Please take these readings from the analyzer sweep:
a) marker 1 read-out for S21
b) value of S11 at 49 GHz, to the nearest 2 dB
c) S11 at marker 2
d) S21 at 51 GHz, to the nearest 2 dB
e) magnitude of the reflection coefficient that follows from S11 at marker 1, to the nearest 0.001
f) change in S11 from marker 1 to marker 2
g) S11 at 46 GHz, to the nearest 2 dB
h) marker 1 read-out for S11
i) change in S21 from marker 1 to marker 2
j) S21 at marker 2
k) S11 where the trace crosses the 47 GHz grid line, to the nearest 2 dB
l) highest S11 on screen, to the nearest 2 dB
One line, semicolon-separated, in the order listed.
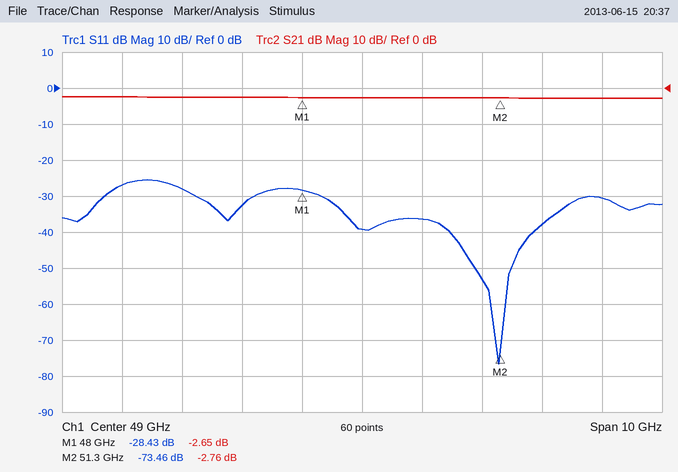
-2.65 dB; -40 dB; -73.46 dB; -2 dB; 0.038; -45.03 dB; -28 dB; -28.43 dB; -0.11 dB; -2.76 dB; -32 dB; -26 dB
